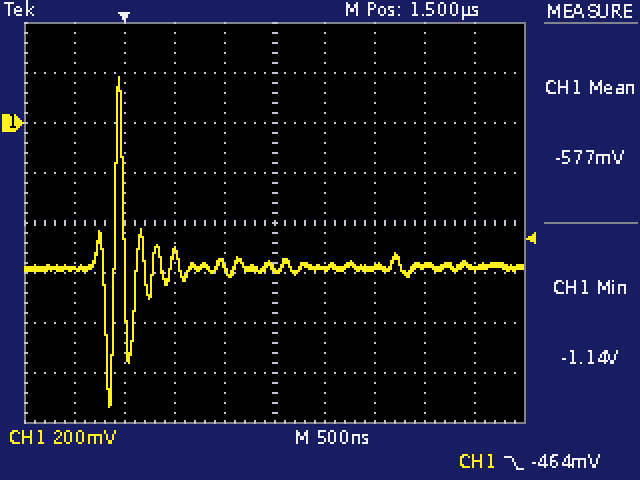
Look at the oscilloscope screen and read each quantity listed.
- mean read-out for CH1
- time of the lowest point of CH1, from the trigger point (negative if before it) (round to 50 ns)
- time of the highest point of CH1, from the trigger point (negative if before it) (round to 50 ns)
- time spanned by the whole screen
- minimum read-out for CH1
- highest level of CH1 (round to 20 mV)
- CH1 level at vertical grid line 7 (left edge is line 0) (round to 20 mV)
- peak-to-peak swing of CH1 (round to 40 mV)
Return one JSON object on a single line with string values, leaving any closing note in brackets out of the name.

{"mean read-out for CH1": "-577 mV", "time of the lowest point of CH1, from the trigger point (negative if before it)": "-150 ns", "time of the highest point of CH1, from the trigger point (negative if before it)": "-50 ns", "time spanned by the whole screen": "5 µs", "minimum read-out for CH1": "-1.14 V", "highest level of CH1": "180 mV", "CH1 level at vertical grid line 7 (left edge is line 0)": "-580 mV", "peak-to-peak swing of CH1": "1.32 V"}
